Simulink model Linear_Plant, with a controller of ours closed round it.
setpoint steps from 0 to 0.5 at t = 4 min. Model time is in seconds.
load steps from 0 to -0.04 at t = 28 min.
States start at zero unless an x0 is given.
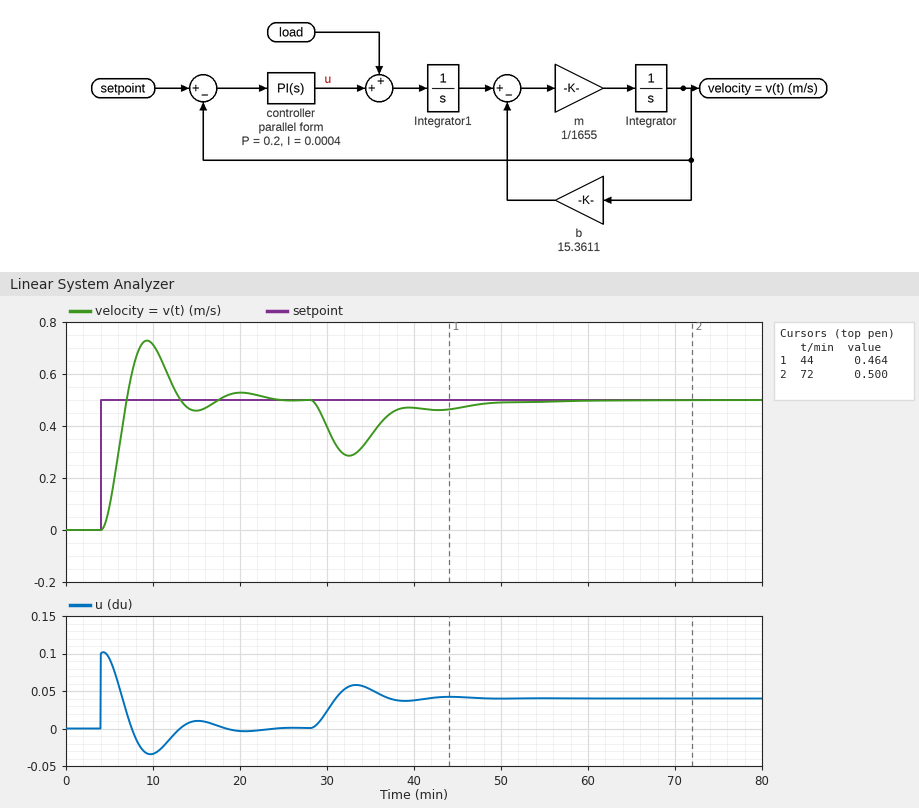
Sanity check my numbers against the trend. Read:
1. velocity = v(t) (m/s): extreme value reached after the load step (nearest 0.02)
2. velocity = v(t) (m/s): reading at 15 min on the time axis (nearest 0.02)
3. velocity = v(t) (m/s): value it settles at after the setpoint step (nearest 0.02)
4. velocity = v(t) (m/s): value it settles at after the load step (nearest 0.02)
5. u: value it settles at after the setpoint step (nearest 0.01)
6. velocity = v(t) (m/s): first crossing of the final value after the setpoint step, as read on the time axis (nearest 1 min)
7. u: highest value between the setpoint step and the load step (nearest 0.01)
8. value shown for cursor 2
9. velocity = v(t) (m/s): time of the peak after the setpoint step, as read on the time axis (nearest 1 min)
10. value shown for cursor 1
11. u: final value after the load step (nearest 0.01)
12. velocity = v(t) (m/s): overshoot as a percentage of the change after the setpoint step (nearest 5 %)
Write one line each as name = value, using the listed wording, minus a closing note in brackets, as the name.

velocity = v(t) (m/s): extreme value reached after the load step = 0.28
velocity = v(t) (m/s): reading at 15 min on the time axis = 0.46
velocity = v(t) (m/s): value it settles at after the setpoint step = 0.50
velocity = v(t) (m/s): value it settles at after the load step = 0.50
u: value it settles at after the setpoint step = 0.00
velocity = v(t) (m/s): first crossing of the final value after the setpoint step, as read on the time axis = 7 min
u: highest value between the setpoint step and the load step = 0.10
value shown for cursor 2 = 0.500
velocity = v(t) (m/s): time of the peak after the setpoint step, as read on the time axis = 9 min
value shown for cursor 1 = 0.464
u: final value after the load step = 0.04
velocity = v(t) (m/s): overshoot as a percentage of the change after the setpoint step = 45 %
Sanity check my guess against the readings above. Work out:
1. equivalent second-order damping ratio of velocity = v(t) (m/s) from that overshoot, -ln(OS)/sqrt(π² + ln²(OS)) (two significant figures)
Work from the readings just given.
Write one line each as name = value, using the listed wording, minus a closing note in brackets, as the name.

equivalent second-order damping ratio of velocity = v(t) (m/s) from that overshoot, -ln(OS)/sqrt(π² + ln²(OS)) = 0.25
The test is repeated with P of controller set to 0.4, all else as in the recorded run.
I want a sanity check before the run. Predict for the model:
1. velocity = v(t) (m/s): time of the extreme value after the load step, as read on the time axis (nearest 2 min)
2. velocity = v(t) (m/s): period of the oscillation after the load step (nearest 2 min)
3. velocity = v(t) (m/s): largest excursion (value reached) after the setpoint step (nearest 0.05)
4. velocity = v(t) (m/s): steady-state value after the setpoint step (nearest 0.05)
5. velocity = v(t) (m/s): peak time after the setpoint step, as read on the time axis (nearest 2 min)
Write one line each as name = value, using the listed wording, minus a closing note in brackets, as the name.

velocity = v(t) (m/s): time of the extreme value after the load step, as read on the time axis = 32 min
velocity = v(t) (m/s): period of the oscillation after the load step = 6 min
velocity = v(t) (m/s): largest excursion (value reached) after the setpoint step = 0.75
velocity = v(t) (m/s): steady-state value after the setpoint step = 0.50
velocity = v(t) (m/s): peak time after the setpoint step, as read on the time axis = 8 min
